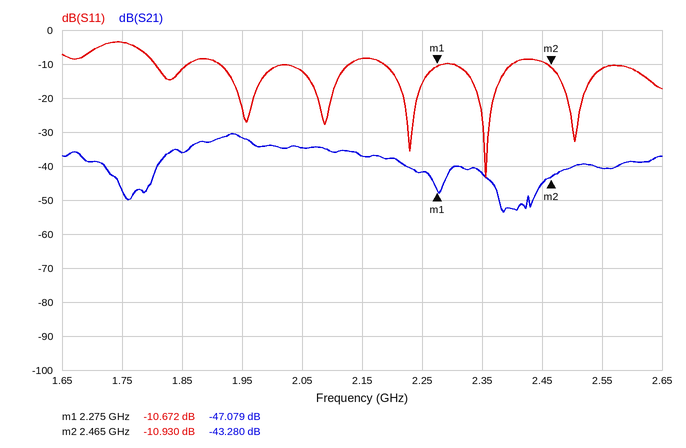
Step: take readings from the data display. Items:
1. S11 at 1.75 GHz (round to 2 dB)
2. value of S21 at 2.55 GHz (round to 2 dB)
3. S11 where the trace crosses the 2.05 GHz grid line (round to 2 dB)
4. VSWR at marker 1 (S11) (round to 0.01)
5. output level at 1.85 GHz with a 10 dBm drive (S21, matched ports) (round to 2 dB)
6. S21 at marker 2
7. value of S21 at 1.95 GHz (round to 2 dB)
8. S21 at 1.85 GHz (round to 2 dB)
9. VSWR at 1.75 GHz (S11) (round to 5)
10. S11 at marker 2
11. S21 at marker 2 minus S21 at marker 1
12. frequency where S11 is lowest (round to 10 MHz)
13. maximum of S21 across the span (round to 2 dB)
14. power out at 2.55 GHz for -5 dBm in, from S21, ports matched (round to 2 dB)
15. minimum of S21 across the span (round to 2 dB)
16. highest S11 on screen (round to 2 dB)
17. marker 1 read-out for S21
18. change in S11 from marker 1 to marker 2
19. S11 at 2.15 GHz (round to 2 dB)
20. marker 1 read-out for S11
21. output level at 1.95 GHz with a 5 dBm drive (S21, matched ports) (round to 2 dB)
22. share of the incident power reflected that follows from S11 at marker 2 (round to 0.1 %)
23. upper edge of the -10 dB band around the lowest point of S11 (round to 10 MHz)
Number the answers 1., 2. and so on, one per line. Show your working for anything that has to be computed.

1. -4 dB
2. -40 dB
3. -12 dB
4. (1 + 0.2927)/(1 − 0.2927) ≈ 1.83
5. 10 dBm + (-36 dB) = -26 dBm
6. -43.280 dB
7. -32 dB
8. -36 dB
9. |Γ| = 10^(-4/20) = 0.6310; VSWR = (1 + 0.6310)/(1 − 0.6310) ≈ 4.42, so 5 to the nearest 5
10. -10.930 dB
11. -43.28 − (-47.079) = 3.799 dB
12. 2.36 GHz
13. -30 dB
14. -5 dBm + (-40 dB) = -46 dBm
15. -54 dB
16. -4 dB
17. -47.079 dB
18. -10.93 − (-10.672) = -0.258 dB
19. -8 dB
20. -10.672 dB
21. 5 dBm + (-32 dB) = -26 dBm
22. 10^(-10.93/10) ≈ 8.1 %
23. 2.40 GHz
